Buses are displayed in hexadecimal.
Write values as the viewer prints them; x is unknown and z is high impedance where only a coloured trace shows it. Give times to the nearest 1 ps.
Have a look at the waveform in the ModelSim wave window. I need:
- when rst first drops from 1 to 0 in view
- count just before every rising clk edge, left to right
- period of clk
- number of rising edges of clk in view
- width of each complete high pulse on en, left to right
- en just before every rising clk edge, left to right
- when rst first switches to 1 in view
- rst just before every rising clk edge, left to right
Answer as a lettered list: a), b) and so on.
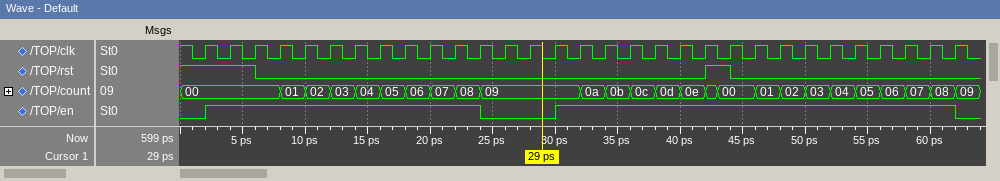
a) 6 ps
b) 00, 00, 00, 00, 01, 02, 03, 04, 05, 06, 07, 08, 09, 09, 09, 09, 0a, 0b, 0c, 0d, 0e, 00, 00, 01, 02, 03, 04, 05, 06, 07, 08
c) 2 ps
d) 31
e) 22 ps, 32 ps
f) 0 1 1 1 1 1 1 1 1 1 1 1 0 0 0 1 1 1 1 1 1 1 1 1 1 1 1 1 1 1 1
g) 42 ps
h) 1 1 1 0 0 0 0 0 0 0 0 0 0 0 0 0 0 0 0 0 0 1 0 0 0 0 0 0 0 0 0
